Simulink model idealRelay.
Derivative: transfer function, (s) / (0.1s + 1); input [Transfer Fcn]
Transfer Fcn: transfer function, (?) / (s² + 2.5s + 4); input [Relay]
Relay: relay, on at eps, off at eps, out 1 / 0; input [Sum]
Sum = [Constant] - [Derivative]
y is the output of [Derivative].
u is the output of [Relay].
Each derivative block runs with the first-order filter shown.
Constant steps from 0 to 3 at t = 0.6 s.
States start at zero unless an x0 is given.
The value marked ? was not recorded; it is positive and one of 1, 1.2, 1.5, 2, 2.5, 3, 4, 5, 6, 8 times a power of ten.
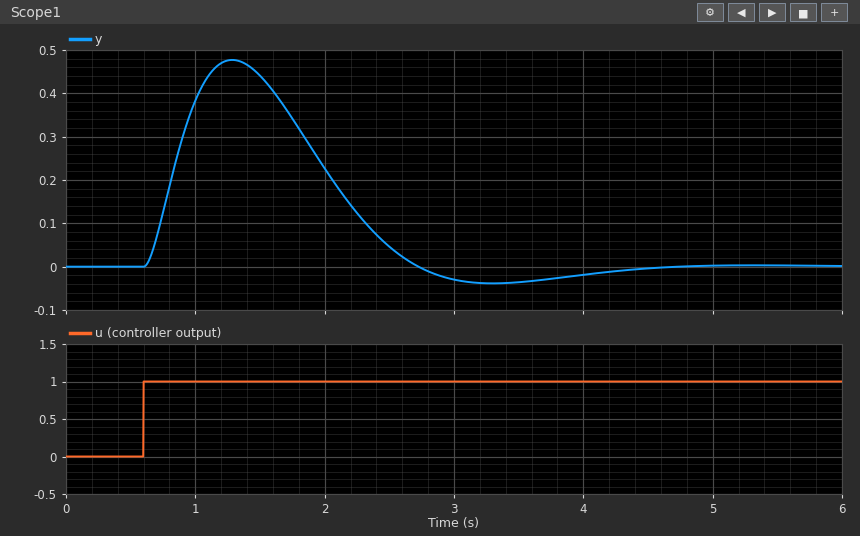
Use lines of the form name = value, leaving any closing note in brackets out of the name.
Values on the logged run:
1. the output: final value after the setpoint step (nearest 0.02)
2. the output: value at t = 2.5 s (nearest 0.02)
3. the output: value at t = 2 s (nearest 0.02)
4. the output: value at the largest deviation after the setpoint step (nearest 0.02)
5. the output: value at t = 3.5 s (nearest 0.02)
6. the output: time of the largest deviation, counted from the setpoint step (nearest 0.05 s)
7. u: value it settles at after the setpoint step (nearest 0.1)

the output: final value after the setpoint step = 0.00
the output: value at t = 2.5 s = 0.04
the output: value at t = 2 s = 0.22
the output: value at the largest deviation after the setpoint step = 0.48
the output: value at t = 3.5 s = -0.04
the output: time of the largest deviation, counted from the setpoint step = 0.70 s
u: value it settles at after the setpoint step = 1.0
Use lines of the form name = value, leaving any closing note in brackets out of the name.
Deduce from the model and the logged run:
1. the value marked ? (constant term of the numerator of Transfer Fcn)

the value marked ? = 2
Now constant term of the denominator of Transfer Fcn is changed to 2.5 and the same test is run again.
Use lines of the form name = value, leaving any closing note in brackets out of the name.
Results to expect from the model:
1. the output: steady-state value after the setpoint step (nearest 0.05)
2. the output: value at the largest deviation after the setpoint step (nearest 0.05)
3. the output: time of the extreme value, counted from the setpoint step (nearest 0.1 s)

the output: steady-state value after the setpoint step = 0.00
the output: value at the largest deviation after the setpoint step = 0.55
the output: time of the extreme value, counted from the setpoint step = 0.8 s
